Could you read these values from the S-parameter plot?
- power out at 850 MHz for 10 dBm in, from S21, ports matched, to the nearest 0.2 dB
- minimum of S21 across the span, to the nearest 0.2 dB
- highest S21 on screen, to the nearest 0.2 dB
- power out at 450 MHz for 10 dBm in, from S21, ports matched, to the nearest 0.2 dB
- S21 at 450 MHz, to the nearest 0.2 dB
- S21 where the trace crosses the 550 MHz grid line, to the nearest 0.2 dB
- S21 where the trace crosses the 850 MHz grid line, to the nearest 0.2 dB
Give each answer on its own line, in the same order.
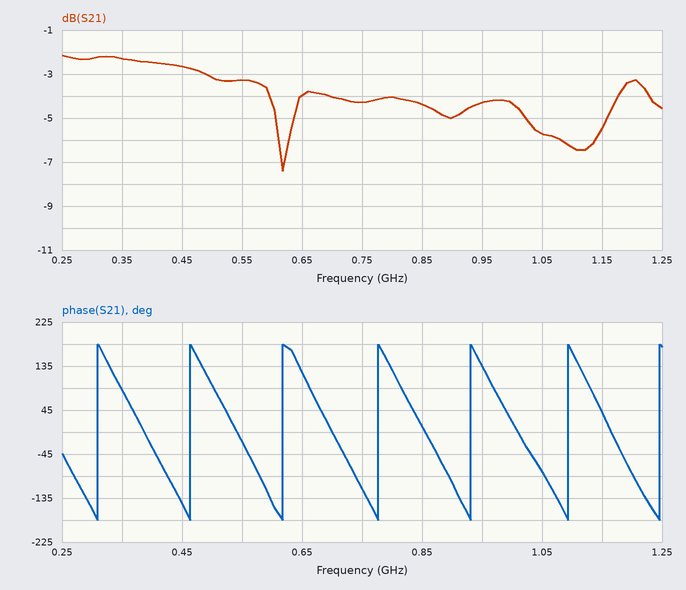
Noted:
5.6 dBm
-7.4 dB
-2.2 dB
7.4 dBm
-2.6 dB
-3.2 dB
-4.4 dB
